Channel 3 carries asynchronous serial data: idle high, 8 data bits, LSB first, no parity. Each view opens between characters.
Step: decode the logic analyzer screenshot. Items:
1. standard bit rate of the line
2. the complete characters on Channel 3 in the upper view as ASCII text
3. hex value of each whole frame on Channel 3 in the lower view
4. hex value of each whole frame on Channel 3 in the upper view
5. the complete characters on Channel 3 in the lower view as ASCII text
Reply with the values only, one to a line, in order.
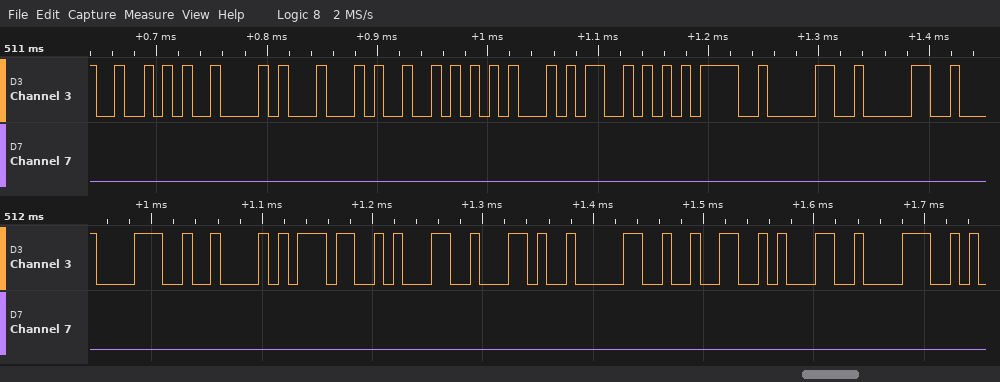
115200 baud
"RBDRES=00"
38, 42, 37, 31, 2C, 30, 32, 31, 38
52, 42, 44, 52, 45, 53, 3D, 30, 30
"8B71,0218"
